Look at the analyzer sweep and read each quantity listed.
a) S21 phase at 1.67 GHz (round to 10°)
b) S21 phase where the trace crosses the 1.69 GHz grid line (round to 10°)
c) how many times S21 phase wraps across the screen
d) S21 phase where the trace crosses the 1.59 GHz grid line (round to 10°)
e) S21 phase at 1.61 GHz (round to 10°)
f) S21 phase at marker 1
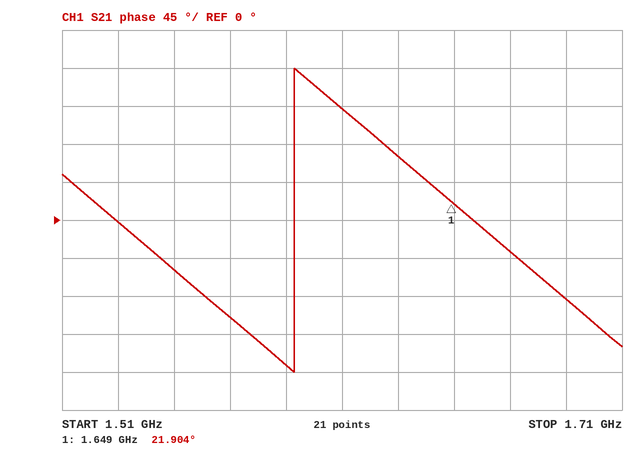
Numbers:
-40°
-90°
1
-170°
130°
21.904°
